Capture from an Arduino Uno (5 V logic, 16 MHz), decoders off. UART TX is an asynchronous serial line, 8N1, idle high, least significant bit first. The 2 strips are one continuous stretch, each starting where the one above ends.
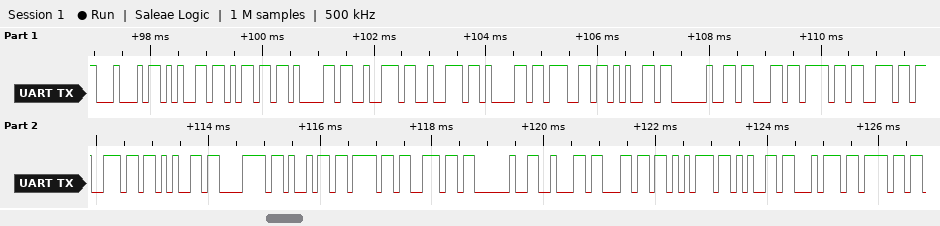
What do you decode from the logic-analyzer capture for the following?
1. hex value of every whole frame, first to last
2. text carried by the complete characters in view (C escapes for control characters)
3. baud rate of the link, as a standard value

44 65 6D 61 72 72 61 67 65 20 63 6F 6E 6E 65 78 69 6F 6E 20 62 6C 75 65 74 6F
"Demarrage connexion blueto"
9600 baud
